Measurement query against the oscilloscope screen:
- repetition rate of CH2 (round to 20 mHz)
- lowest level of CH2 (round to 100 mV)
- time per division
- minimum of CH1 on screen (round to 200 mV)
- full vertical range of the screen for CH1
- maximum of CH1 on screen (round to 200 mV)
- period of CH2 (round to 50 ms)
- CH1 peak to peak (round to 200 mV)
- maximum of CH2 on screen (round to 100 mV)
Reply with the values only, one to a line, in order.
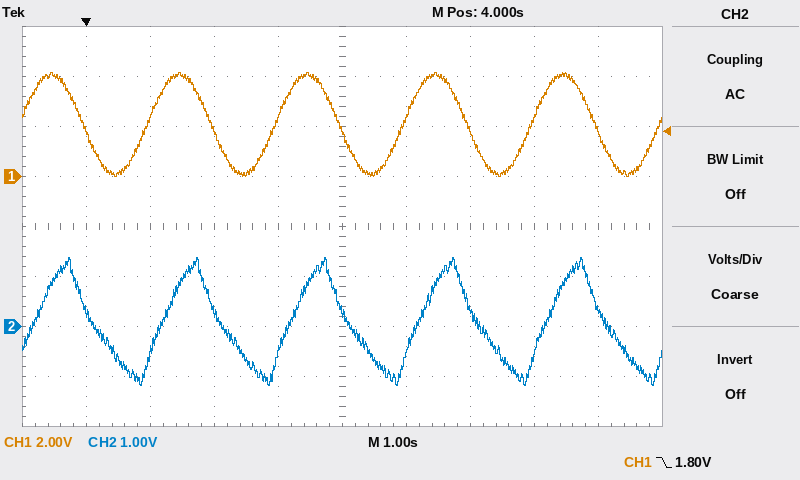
500 mHz
-1.2 V
1 s
0.0 V
16 V
4.2 V
2.00 s
4.2 V
1.4 V
